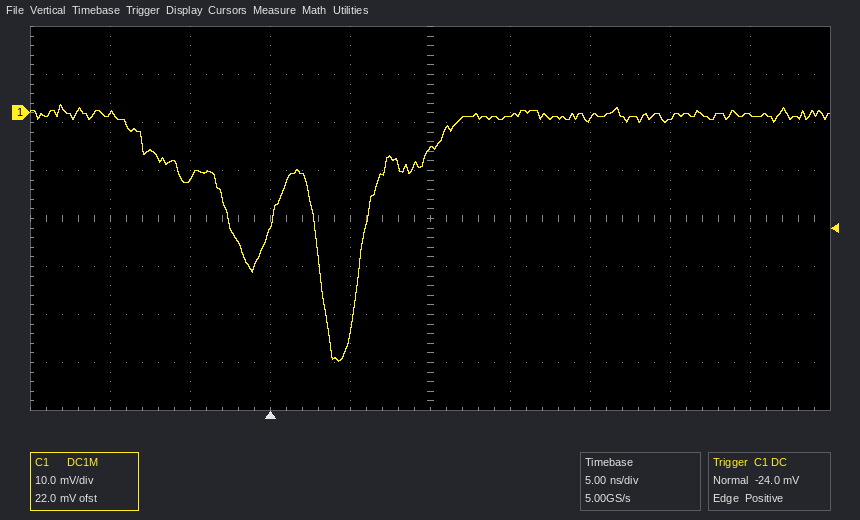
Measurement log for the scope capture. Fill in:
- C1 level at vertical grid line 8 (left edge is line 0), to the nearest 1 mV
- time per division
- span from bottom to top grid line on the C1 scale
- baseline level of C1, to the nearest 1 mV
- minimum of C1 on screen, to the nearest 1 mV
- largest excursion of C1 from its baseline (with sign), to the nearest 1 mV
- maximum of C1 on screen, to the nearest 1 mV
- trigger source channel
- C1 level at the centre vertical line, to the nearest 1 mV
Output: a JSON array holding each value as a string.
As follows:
["-1 mV", "5 ns", "80 mV", "-1 mV", "-52 mV", "-51 mV", "2 mV", "C1", "-8 mV"]
